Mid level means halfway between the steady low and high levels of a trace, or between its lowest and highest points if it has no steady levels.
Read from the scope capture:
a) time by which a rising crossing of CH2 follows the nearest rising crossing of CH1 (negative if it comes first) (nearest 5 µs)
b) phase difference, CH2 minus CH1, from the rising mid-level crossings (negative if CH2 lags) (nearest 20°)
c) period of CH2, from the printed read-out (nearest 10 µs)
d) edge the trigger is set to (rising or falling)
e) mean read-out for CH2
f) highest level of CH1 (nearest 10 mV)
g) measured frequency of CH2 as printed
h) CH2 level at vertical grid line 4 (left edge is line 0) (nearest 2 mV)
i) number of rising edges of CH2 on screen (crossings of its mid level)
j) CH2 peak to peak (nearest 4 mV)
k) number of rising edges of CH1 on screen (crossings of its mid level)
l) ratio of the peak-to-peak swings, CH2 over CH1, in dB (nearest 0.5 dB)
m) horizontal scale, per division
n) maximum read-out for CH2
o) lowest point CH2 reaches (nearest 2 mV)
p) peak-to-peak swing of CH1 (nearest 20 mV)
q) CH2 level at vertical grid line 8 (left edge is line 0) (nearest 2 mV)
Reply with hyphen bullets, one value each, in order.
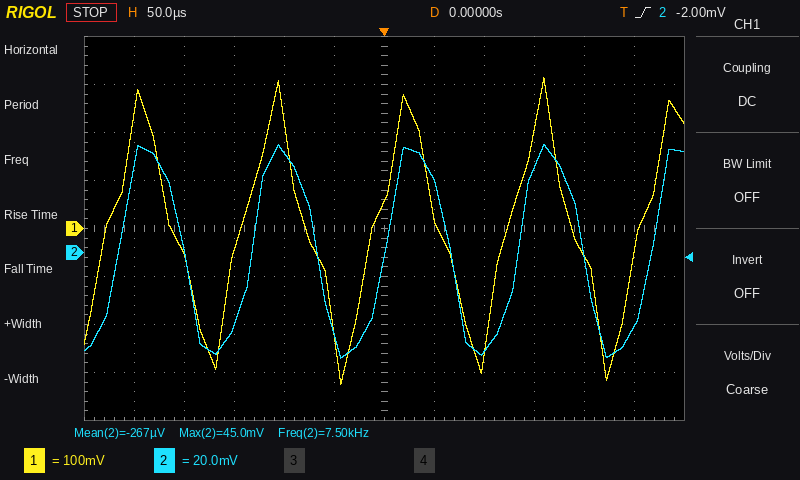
- +15 µs
- -40°
- 130 µs
- rising
- -267 µV
- 310 mV
- 7.50 kHz
- 42 mV
- 5
- 88 mV
- 5
- -17.0 dB
- 50 µs
- 45.0 mV
- -44 mV
- 640 mV
- -42 mV
